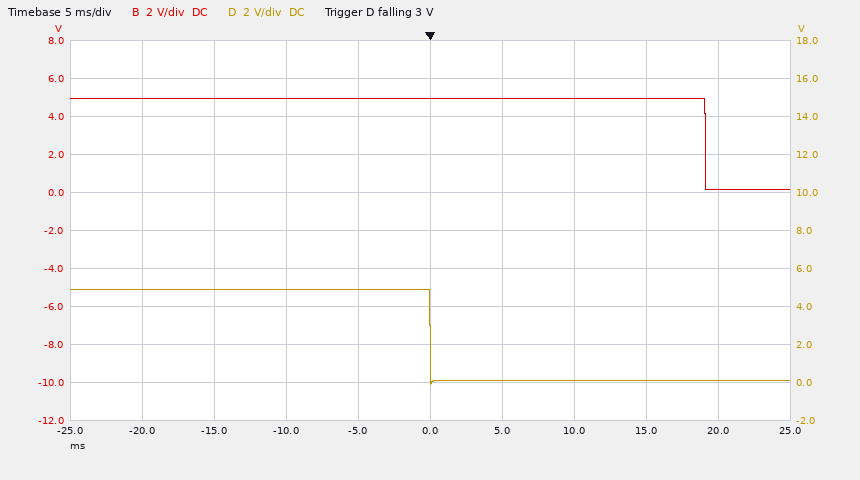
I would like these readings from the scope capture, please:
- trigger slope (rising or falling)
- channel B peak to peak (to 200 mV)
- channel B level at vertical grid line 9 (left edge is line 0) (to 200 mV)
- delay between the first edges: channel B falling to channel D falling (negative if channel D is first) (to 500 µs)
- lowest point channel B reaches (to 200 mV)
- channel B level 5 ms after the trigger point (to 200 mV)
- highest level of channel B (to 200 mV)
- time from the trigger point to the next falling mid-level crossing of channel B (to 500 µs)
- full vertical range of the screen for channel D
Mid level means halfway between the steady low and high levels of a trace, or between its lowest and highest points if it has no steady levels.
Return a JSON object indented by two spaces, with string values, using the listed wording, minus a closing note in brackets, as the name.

{
  "trigger slope": "falling",
  "channel B peak to peak": "4.8 V",
  "channel B level at vertical grid line 9 (left edge is line 0)": "200 mV",
  "delay between the first edges: channel B falling to channel D falling (negative if channel D is first)": "-19.0 ms",
  "lowest point channel B reaches": "200 mV",
  "channel B level 5 ms after the trigger point": "5.0 V",
  "highest level of channel B": "5.0 V",
  "time from the trigger point to the next falling mid-level crossing of channel B": "19.0 ms",
  "full vertical range of the screen for channel D": "20 V"
}
